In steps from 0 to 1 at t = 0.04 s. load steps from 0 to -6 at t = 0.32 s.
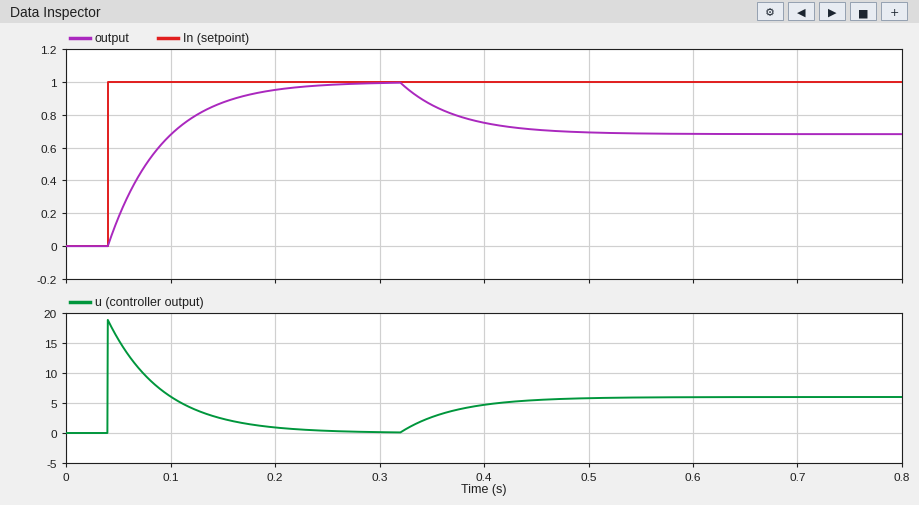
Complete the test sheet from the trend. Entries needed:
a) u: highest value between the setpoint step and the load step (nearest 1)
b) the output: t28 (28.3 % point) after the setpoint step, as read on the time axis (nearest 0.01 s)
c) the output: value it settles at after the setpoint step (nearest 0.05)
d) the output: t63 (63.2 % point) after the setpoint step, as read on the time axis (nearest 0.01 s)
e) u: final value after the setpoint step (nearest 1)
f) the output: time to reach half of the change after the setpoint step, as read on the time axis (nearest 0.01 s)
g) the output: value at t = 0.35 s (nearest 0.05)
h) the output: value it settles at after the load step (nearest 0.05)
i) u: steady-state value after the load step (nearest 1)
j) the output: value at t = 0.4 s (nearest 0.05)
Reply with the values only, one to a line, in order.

19
0.06 s
1.00
0.09 s
0
0.08 s
0.85
0.70
6
0.75
